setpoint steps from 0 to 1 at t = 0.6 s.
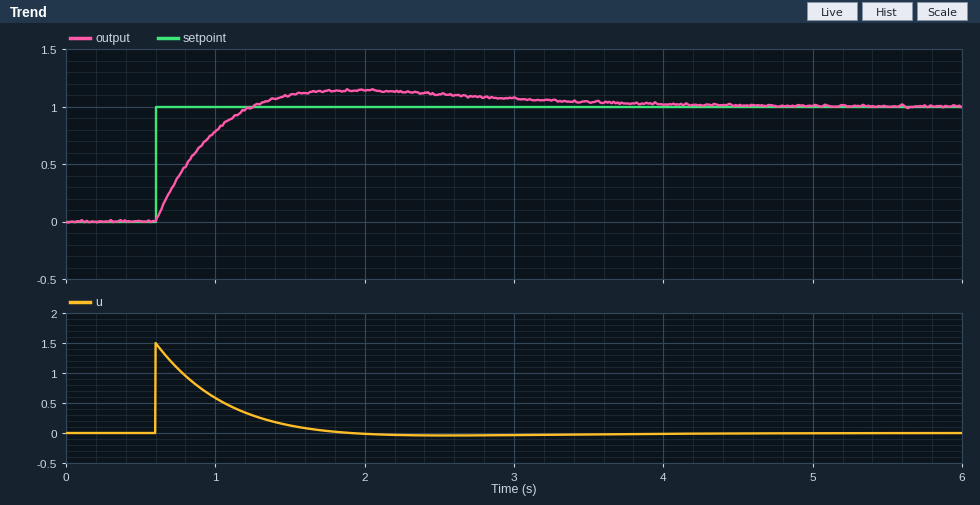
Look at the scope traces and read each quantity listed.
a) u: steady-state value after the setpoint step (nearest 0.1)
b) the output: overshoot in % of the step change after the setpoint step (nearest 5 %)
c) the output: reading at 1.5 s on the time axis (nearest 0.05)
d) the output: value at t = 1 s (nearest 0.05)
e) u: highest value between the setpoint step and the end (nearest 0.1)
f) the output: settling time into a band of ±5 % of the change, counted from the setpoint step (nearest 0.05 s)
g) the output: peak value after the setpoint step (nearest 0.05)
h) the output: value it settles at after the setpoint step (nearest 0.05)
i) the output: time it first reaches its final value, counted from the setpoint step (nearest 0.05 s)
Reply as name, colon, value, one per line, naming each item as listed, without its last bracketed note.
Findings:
u: steady-state value after the setpoint step: 0.0
the output: overshoot in % of the step change after the setpoint step: 15 %
the output: reading at 1.5 s on the time axis: 1.10
the output: value at t = 1 s: 0.80
u: highest value between the setpoint step and the end: 1.5
the output: settling time into a band of ±5 % of the change, counted from the setpoint step: 2.70 s
the output: peak value after the setpoint step: 1.15
the output: value it settles at after the setpoint step: 1.00
the output: time it first reaches its final value, counted from the setpoint step: 0.65 s
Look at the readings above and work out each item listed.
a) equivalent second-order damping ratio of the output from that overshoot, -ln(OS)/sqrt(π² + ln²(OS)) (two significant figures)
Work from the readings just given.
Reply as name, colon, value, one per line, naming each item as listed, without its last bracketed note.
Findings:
equivalent second-order damping ratio of the output from that overshoot, -ln(OS)/sqrt(π² + ln²(OS)): 0.52
